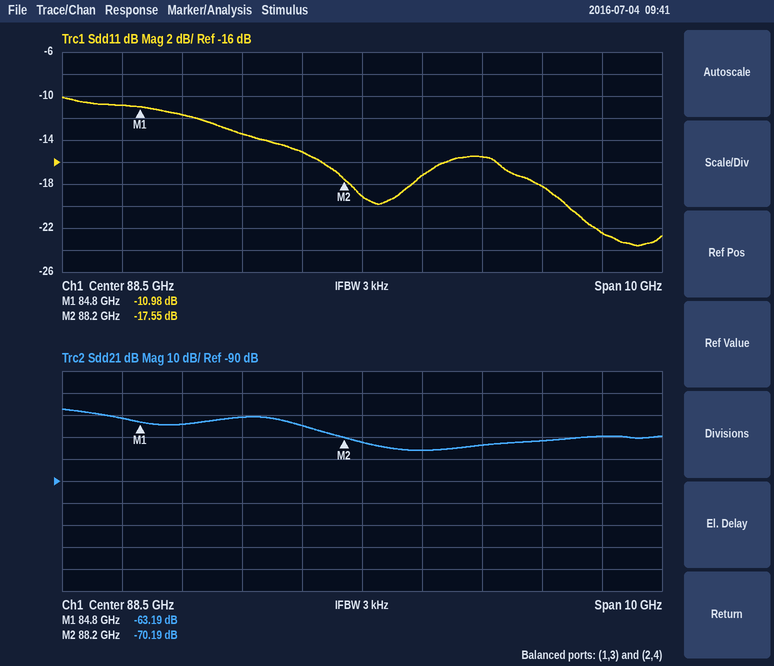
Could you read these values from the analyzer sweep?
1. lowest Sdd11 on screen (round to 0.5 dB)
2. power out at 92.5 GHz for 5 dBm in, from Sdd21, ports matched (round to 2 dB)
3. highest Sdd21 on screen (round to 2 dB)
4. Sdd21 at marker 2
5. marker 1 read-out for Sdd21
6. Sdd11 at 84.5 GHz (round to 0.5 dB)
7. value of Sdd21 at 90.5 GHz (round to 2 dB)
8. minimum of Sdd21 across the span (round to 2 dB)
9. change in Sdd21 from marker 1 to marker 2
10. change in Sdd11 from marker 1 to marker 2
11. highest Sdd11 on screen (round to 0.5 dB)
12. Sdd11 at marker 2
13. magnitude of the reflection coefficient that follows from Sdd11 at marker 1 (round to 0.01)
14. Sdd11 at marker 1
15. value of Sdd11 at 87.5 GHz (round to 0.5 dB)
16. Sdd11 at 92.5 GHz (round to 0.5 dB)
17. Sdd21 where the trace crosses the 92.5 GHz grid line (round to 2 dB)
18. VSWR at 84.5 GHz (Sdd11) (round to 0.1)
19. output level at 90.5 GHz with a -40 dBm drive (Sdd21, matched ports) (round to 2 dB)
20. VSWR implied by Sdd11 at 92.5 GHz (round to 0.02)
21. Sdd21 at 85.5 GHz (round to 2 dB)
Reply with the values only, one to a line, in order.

-23.5 dB
-64 dBm
-58 dB
-70.19 dB
-63.19 dB
-11.0 dB
-74 dB
-76 dB
-7.00 dB
-6.57 dB
-10.0 dB
-17.55 dB
0.28
-10.98 dB
-15.0 dB
-22.5 dB
-70 dB
1.8
-114 dBm
1.16
-64 dB
